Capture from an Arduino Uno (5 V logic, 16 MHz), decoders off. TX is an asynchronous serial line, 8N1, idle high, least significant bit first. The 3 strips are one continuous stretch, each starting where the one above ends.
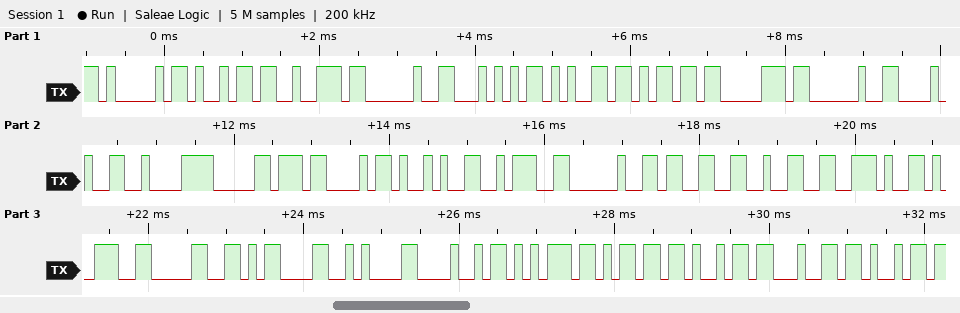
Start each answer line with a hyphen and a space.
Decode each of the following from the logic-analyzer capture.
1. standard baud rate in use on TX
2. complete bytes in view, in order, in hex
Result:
- 9600 baud
- 0x41 0x69 0x72 0x20 0x54 0x65 0x6D 0x70 0x20 0x28 0xC2 0xB0 0x43 0x29 0x3A 0x20 0x33 0x32 0x2E 0x39 0x30 0x0D 0x0A 0x48 0x75 0x6D 0x69 0x64 0x69
